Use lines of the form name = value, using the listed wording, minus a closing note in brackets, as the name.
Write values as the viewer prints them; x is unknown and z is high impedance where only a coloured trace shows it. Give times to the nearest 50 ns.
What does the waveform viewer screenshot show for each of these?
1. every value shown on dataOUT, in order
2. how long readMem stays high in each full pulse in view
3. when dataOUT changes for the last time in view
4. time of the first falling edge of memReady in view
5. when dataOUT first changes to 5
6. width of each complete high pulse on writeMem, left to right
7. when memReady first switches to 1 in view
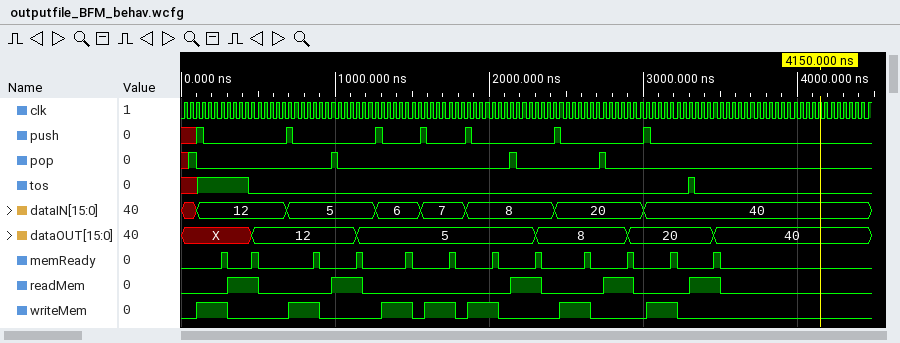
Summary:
every value shown on dataOUT, in order = X, 12, 5, 8, 20, 40
how long readMem stays high in each full pulse in view = 200 ns, 200 ns, 200 ns, 200 ns, 200 ns
when dataOUT changes for the last time in view = 3450 ns
time of the first falling edge of memReady in view = 300 ns
when dataOUT first changes to 5 = 1150 ns
width of each complete high pulse on writeMem, left to right = 200 ns, 200 ns, 200 ns, 200 ns, 200 ns, 200 ns, 200 ns
when memReady first switches to 1 in view = 250 ns
